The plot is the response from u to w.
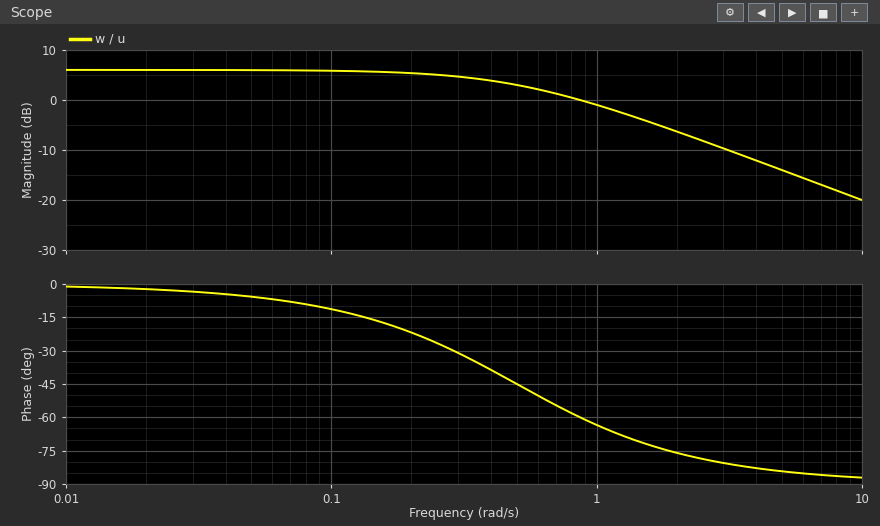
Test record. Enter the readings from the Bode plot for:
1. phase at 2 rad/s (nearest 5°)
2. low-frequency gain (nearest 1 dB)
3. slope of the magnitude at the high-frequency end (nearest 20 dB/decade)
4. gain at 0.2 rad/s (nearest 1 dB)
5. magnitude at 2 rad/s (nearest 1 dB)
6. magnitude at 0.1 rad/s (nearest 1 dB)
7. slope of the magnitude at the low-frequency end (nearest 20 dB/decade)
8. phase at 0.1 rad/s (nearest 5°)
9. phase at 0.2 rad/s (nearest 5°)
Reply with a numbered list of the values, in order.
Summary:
1. -75°
2. 6 dB
3. -20 dB/decade
4. 5 dB
5. -6 dB
6. 6 dB
7. 0 dB/decade
8. -10°
9. -20°
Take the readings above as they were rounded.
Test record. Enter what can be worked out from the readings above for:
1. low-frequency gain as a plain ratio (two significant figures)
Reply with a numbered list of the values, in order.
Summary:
1. 2.0
